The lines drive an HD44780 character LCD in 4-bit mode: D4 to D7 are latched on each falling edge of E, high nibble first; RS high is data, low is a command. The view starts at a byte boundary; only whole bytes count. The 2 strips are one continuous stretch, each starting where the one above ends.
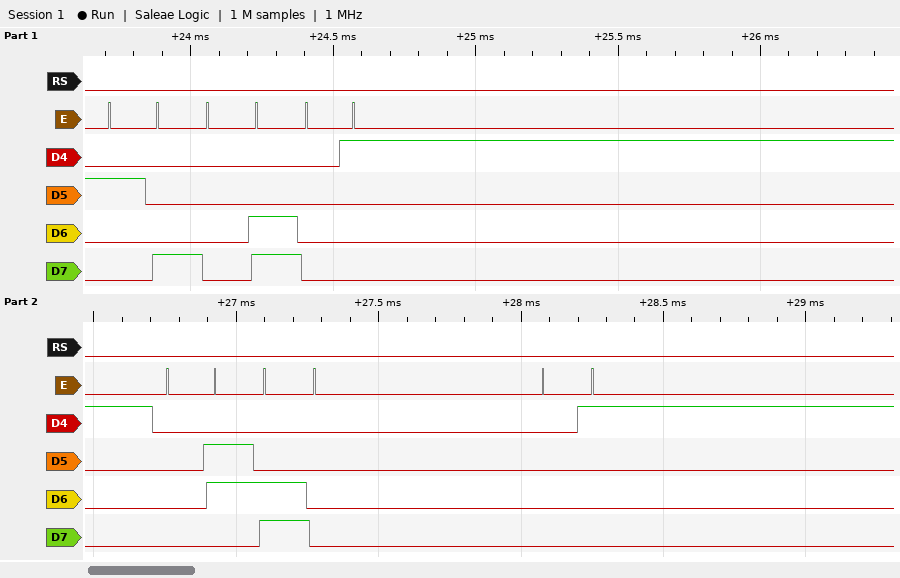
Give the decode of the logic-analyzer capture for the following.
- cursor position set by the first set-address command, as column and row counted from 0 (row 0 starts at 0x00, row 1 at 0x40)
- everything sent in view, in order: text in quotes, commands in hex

column 0, row 1
0x28 0x0C 0x01 0x06 0xC0 0x01
